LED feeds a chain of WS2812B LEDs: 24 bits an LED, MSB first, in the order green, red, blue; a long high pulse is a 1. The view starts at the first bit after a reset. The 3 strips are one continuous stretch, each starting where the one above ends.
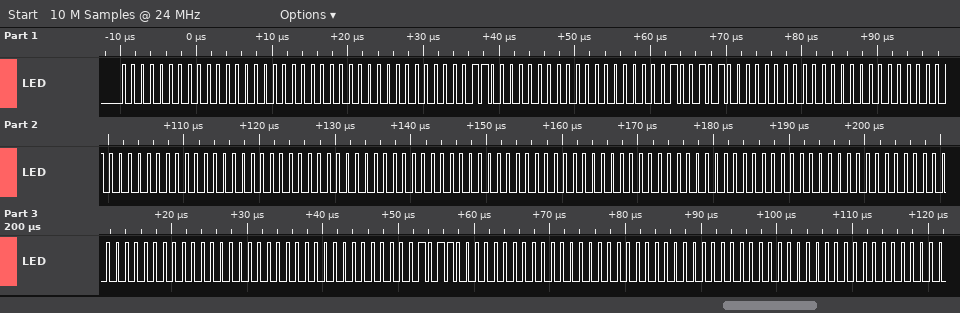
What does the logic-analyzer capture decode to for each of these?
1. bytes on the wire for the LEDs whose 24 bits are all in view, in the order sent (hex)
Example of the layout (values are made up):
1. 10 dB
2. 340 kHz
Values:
1. 00 00 00 00 06 00 00 25 00 00 00 00 00 00 00 00 00 00 00 00 00 00 00 00 00 00 2C 00 00 00 00 00 00
